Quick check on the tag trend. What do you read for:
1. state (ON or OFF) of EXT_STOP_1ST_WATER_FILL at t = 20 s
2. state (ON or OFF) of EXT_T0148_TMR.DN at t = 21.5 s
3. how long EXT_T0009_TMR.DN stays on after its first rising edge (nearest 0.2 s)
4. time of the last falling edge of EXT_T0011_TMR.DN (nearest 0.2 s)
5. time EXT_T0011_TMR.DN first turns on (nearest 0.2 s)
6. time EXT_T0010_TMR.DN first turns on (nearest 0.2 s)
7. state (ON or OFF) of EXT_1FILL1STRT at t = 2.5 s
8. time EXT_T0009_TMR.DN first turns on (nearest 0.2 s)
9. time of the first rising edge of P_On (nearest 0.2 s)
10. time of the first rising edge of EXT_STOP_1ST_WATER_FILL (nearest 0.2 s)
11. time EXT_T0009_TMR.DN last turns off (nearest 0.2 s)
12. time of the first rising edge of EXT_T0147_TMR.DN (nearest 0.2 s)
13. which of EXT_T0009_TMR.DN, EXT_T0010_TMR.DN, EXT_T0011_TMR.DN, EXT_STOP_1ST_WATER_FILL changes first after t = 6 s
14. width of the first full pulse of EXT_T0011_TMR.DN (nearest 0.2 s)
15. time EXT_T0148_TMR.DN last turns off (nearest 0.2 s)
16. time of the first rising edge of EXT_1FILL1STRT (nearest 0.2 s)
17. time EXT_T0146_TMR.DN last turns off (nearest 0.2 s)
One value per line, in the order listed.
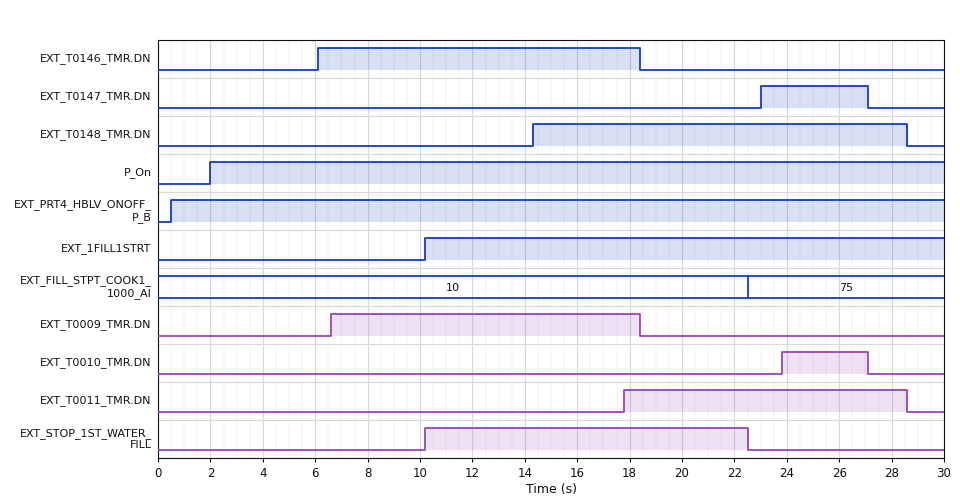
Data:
ON
ON
11.8 s
28.6 s
17.8 s
23.8 s
OFF
6.6 s
2.0 s
10.2 s
18.4 s
23.0 s
EXT_T0009_TMR.DN
10.8 s
28.6 s
10.2 s
18.4 s
